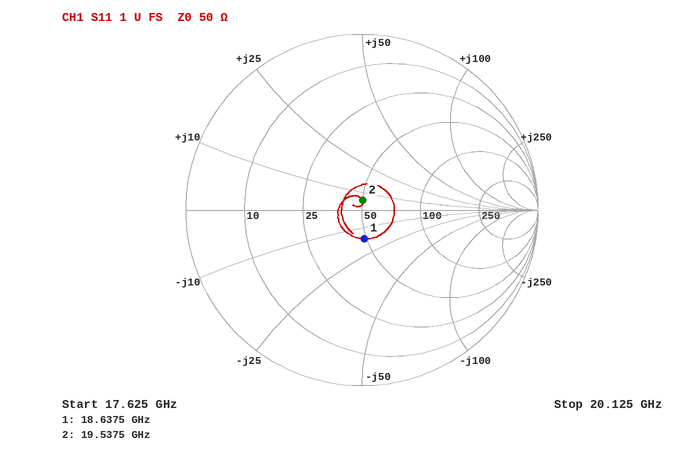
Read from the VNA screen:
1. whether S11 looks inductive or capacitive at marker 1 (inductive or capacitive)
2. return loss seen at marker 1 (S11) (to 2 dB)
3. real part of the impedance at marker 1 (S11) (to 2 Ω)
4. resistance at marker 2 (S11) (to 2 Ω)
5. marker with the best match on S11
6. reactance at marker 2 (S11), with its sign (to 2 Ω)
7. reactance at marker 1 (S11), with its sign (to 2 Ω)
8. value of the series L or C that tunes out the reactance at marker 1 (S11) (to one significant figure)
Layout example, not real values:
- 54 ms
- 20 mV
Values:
- capacitive
- 16 dB
- 48 Ω
- 50 Ω
- marker 2
- +6 Ω
- -16 Ω
- 100 pH
